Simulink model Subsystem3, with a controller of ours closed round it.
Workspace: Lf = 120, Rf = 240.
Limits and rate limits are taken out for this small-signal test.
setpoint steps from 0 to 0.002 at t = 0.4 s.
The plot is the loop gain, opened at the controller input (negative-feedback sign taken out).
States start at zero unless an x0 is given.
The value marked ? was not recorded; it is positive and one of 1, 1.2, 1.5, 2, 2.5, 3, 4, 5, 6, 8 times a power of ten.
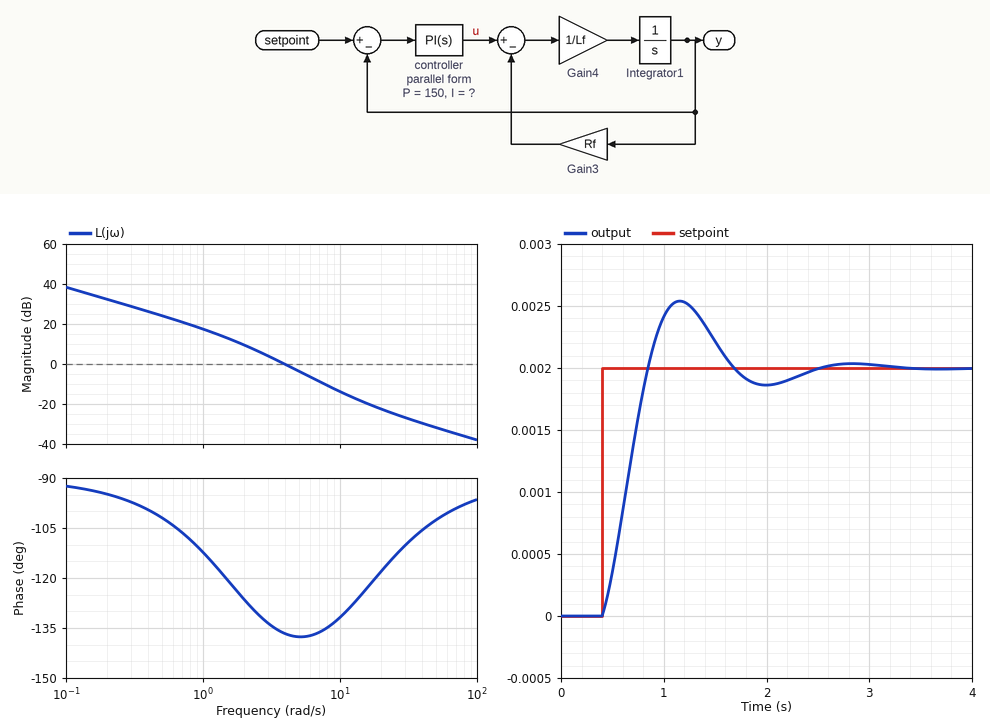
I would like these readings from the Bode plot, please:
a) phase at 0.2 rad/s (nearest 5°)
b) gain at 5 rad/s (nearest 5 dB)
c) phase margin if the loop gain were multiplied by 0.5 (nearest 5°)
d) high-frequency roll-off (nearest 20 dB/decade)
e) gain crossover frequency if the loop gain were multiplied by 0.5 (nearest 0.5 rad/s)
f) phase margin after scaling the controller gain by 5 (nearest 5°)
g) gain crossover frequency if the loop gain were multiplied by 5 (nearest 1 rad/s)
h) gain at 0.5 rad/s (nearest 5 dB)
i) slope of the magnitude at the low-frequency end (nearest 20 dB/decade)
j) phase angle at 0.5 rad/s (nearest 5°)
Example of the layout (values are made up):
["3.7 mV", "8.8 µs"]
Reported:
["-95°", "-5 dB", "50°", "-20 dB/decade", "2.5 rad/s", "50°", "10 rad/s", "25 dB", "-20 dB/decade", "-100°"]
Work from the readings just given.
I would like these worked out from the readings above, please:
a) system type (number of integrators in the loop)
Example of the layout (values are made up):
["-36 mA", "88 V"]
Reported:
["1"]
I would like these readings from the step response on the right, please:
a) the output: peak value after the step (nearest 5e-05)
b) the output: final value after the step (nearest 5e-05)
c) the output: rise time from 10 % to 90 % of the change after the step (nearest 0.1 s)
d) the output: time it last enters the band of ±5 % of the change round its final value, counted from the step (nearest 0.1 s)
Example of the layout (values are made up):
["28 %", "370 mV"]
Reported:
["0.00255", "0.00200", "0.3 s", "1.8 s"]
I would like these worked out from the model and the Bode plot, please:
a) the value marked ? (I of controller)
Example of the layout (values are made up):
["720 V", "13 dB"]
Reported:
["2000"]
